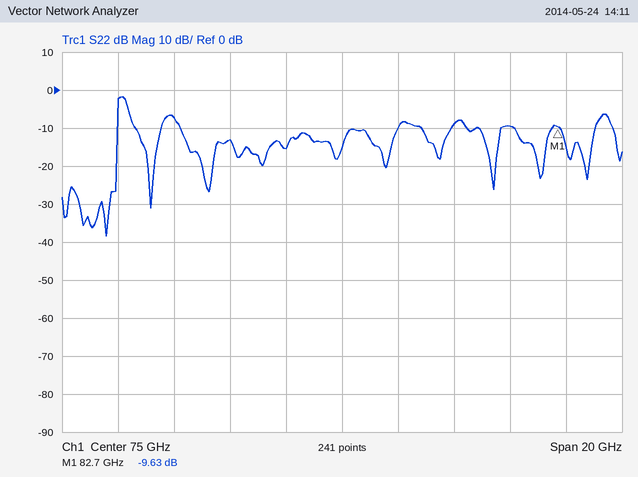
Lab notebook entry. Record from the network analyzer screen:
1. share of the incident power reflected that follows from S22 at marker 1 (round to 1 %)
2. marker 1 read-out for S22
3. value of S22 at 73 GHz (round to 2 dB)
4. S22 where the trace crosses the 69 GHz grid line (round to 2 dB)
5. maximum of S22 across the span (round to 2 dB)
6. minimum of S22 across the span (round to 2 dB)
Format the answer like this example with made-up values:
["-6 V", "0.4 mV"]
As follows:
["11 %", "-9.63 dB", "-16 dB", "-8 dB", "-2 dB", "-38 dB"]
